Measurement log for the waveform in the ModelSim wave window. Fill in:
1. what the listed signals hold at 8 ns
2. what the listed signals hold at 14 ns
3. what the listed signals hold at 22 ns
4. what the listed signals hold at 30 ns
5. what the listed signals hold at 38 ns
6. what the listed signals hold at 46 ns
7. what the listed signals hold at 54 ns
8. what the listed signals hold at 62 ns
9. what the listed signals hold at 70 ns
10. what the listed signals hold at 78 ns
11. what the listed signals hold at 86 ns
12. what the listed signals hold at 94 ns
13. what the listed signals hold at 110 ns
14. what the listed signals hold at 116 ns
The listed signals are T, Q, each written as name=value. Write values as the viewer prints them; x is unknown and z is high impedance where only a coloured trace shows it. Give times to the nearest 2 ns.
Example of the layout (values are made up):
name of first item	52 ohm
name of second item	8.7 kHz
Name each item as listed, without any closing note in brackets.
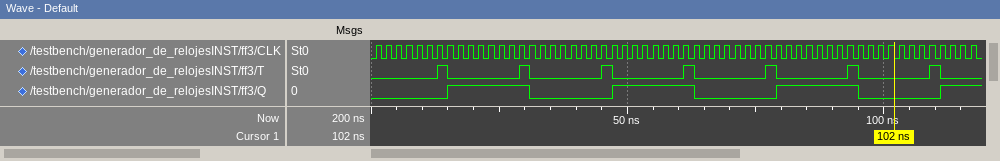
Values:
what the listed signals hold at 8 ns	T=0, Q=0
what the listed signals hold at 14 ns	T=1, Q=0
what the listed signals hold at 22 ns	T=0, Q=1
what the listed signals hold at 30 ns	T=1, Q=1
what the listed signals hold at 38 ns	T=0, Q=0
what the listed signals hold at 46 ns	T=1, Q=0
what the listed signals hold at 54 ns	T=0, Q=1
what the listed signals hold at 62 ns	T=1, Q=1
what the listed signals hold at 70 ns	T=0, Q=0
what the listed signals hold at 78 ns	T=1, Q=0
what the listed signals hold at 86 ns	T=0, Q=1
what the listed signals hold at 94 ns	T=1, Q=1
what the listed signals hold at 110 ns	T=1, Q=0
what the listed signals hold at 116 ns	T=0, Q=1
